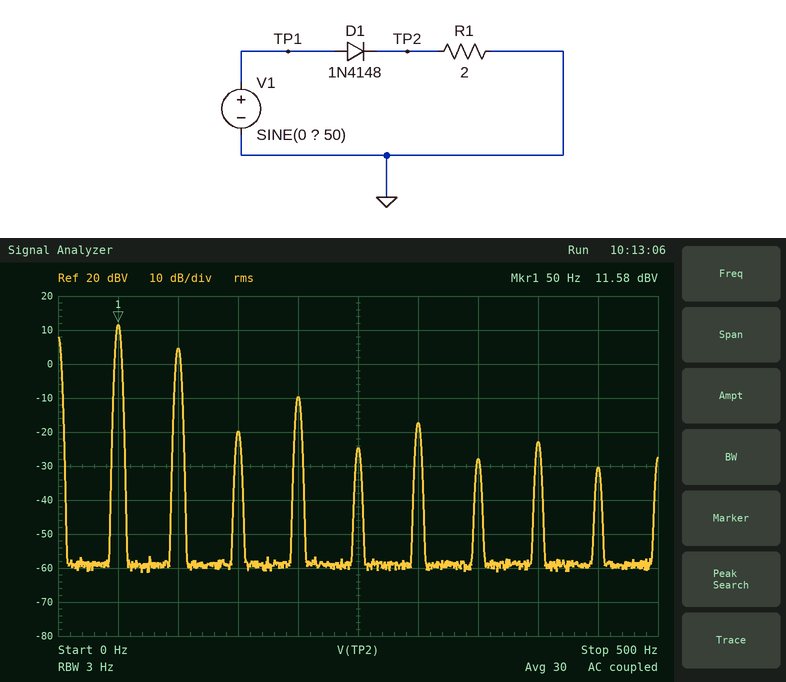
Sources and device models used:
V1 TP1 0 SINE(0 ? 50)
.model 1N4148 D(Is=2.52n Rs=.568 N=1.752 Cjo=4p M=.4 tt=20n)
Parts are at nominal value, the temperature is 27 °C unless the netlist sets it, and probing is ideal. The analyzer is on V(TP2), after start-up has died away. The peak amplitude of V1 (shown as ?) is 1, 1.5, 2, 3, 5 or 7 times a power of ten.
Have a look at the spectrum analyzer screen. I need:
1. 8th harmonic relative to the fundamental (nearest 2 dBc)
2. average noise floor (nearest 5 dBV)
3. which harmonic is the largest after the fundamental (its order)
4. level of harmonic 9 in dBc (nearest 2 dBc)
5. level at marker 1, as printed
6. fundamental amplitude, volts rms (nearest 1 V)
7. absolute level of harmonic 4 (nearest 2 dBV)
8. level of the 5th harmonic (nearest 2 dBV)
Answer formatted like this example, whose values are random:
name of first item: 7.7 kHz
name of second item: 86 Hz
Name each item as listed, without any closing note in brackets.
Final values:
8th harmonic relative to the fundamental: -34 dBc
average noise floor: -60 dBV
which harmonic is the largest after the fundamental: 2
level of harmonic 9 in dBc: -42 dBc
level at marker 1, as printed: 11.58 dBV
fundamental amplitude, volts rms: 4 V
absolute level of harmonic 4: -10 dBV
level of the 5th harmonic: -24 dBV
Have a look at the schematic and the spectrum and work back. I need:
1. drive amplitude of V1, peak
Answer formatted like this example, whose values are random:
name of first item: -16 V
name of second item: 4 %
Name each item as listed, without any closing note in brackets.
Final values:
drive amplitude of V1, peak: 15 V
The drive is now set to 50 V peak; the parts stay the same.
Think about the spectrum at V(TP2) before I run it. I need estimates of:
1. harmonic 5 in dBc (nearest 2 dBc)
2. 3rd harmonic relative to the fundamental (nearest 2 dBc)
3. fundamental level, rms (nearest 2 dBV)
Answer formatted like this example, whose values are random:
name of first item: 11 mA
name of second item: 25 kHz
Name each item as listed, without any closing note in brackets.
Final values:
harmonic 5 in dBc: -46 dBc
3rd harmonic relative to the fundamental: -42 dBc
fundamental level, rms: 22 dBV
